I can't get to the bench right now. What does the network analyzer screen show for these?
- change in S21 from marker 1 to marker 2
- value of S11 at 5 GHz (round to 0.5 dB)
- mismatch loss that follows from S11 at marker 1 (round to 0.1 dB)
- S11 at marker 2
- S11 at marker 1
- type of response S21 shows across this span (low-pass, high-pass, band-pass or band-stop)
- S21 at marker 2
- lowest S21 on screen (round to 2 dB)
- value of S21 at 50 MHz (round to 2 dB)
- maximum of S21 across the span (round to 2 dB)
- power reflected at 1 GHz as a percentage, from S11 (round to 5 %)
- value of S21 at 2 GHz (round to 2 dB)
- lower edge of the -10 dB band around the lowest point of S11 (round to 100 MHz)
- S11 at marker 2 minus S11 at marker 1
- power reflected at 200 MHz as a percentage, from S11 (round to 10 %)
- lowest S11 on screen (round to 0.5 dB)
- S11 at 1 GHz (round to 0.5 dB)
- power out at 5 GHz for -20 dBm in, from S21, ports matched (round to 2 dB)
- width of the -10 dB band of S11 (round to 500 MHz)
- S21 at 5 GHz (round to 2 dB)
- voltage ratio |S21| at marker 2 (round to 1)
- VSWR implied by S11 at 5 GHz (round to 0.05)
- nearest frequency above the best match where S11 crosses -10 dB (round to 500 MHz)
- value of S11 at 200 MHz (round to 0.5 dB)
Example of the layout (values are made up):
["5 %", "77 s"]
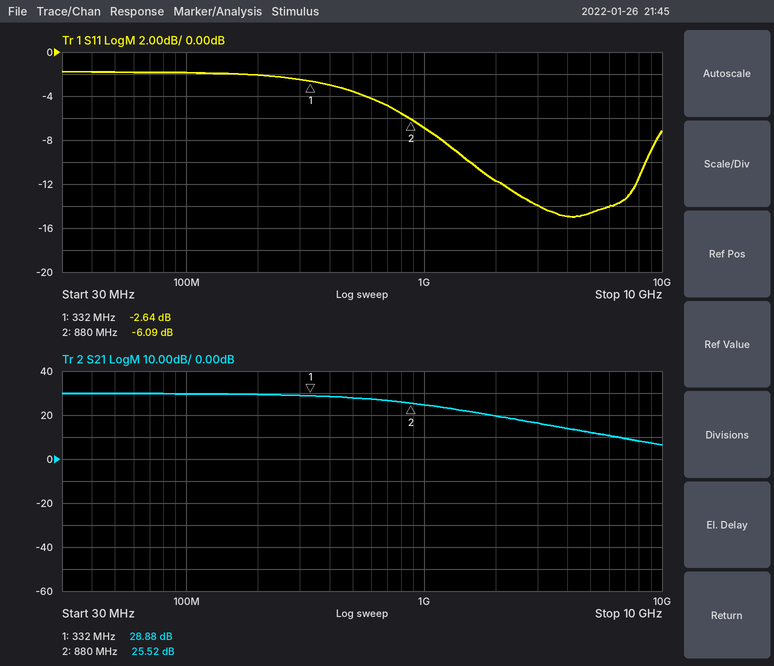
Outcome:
["-3.36 dB", "-14.5 dB", "3.4 dB", "-6.09 dB", "-2.64 dB", "low-pass", "25.52 dB", "6 dB", "30 dB", "30 dB", "20 %", "20 dB", "1.6 GHz", "-3.45 dB", "60 %", "-15.0 dB", "-7.0 dB", "-8 dBm", "7.0 GHz", "12 dB", "19", "1.45", "8.5 GHz", "-2.0 dB"]
